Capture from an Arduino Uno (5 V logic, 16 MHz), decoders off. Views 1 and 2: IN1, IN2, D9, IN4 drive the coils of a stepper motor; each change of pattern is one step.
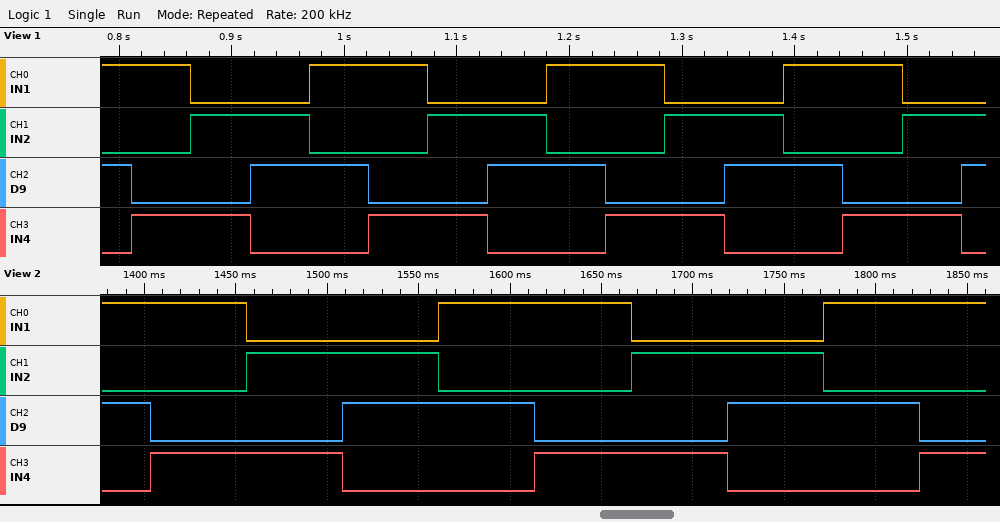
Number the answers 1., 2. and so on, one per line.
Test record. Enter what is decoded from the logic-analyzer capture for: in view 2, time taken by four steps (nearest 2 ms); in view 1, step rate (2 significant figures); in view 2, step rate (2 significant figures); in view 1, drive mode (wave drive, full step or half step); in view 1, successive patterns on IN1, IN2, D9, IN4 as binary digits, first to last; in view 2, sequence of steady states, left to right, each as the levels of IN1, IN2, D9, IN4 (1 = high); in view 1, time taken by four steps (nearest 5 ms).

1. 210 ms
2. 19 steps/s
3. 19 steps/s
4. full step
5. 1010 1001 0101 0110 1010 1001 0101 0110 1010 1001 0101 0110 1010 1001 0101 0110
6. 1010 1001 0101 0110 1010 1001 0101 0110 1010 1001
7. 210 ms
